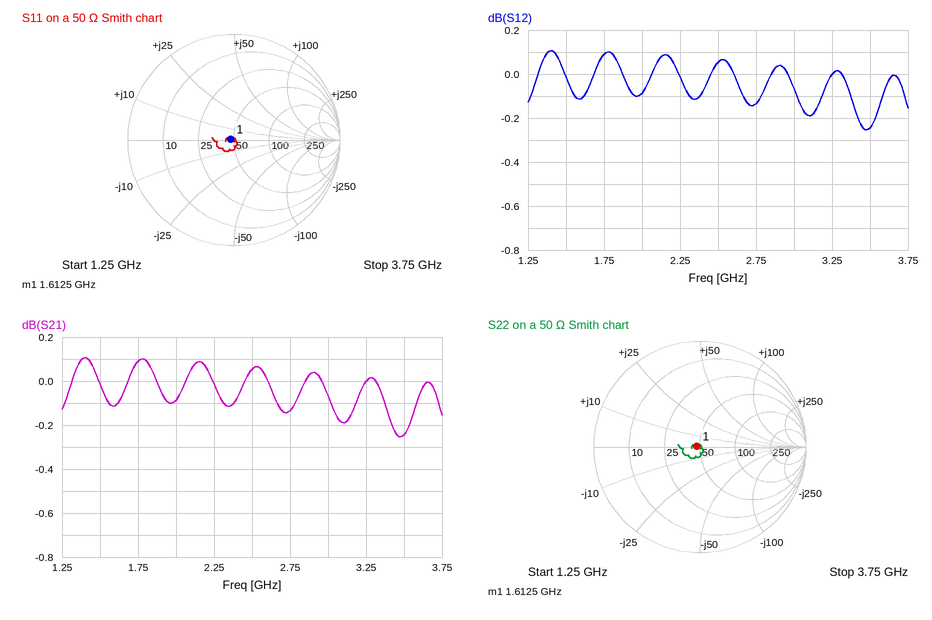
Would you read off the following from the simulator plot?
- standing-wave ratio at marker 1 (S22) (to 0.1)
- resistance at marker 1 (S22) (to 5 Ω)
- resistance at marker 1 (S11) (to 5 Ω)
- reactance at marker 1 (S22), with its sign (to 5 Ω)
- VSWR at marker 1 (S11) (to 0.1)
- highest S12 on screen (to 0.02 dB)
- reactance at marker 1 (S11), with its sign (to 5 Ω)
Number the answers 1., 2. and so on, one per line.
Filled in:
1. 1.1
2. 45 Ω
3. 45 Ω
4. 0 Ω
5. 1.1
6. 0.10 dB
7. 0 Ω
